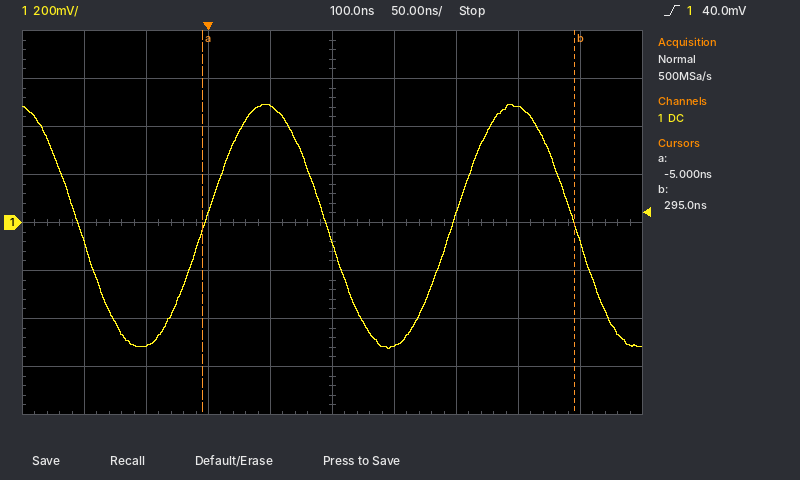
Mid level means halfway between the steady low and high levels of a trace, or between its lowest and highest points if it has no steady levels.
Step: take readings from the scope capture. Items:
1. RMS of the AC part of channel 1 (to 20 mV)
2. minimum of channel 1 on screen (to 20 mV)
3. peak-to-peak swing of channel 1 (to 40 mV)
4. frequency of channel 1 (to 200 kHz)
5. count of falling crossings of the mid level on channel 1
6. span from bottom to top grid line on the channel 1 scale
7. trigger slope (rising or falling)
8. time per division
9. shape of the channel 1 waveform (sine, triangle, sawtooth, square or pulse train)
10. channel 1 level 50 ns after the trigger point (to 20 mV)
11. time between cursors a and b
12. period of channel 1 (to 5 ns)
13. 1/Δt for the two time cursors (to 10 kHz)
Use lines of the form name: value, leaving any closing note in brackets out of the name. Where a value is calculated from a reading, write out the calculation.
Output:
RMS of the AC part of channel 1: 1.00 V / (2√2) ≈ 354 mV, so 360 mV to the nearest 20 mV
minimum of channel 1 on screen: -520 mV
peak-to-peak swing of channel 1: 1.00 V
frequency of channel 1: 1 / 200 ns ≈ 5.0 MHz
count of falling crossings of the mid level on channel 1: 3
span from bottom to top grid line on the channel 1 scale: 1.6 V
trigger slope: rising
time per division: 50 ns
shape of the channel 1 waveform: sine
channel 1 level 50 ns after the trigger point: 480 mV
time between cursors a and b: 295 ns − (-5 ns) = 300 ns
period of channel 1: 200 ns
1/Δt for the two time cursors: 1 / 300 ns ≈ 3.33 MHz
